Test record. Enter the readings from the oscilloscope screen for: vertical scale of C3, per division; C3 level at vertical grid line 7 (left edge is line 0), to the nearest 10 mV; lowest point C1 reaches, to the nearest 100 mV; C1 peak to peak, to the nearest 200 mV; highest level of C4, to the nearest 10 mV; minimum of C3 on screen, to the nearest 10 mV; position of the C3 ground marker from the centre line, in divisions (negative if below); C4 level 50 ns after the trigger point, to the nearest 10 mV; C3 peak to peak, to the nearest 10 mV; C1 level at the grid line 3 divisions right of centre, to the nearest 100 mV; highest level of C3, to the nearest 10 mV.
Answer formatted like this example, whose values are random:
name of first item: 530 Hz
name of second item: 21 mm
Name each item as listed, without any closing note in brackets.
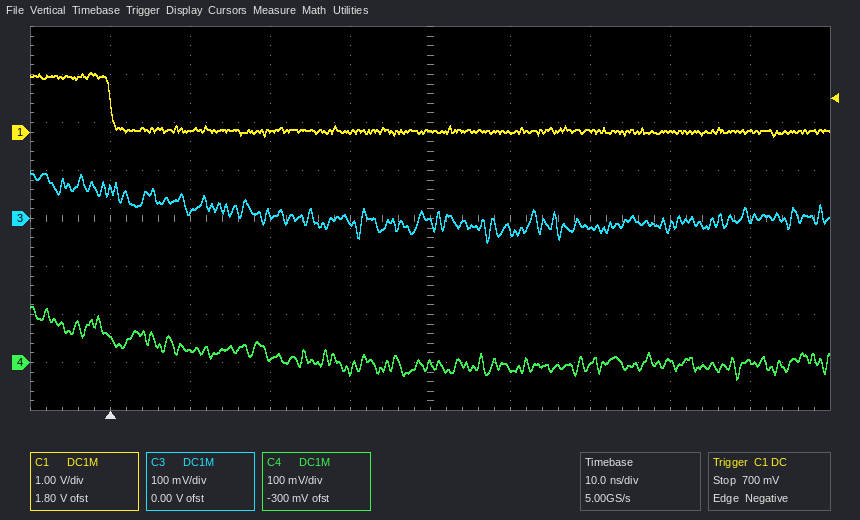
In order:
vertical scale of C3, per division: 100 mV
C3 level at vertical grid line 7 (left edge is line 0), to the nearest 10 mV: -20 mV
lowest point C1 reaches, to the nearest 100 mV: -100 mV
C1 peak to peak, to the nearest 200 mV: 1.4 V
highest level of C4, to the nearest 10 mV: 120 mV
minimum of C3 on screen, to the nearest 10 mV: -50 mV
position of the C3 ground marker from the centre line, in divisions: 0.0 div
C4 level 50 ns after the trigger point, to the nearest 10 mV: -10 mV
C3 peak to peak, to the nearest 10 mV: 150 mV
C1 level at the grid line 3 divisions right of centre, to the nearest 100 mV: 0.0 V
highest level of C3, to the nearest 10 mV: 100 mV
